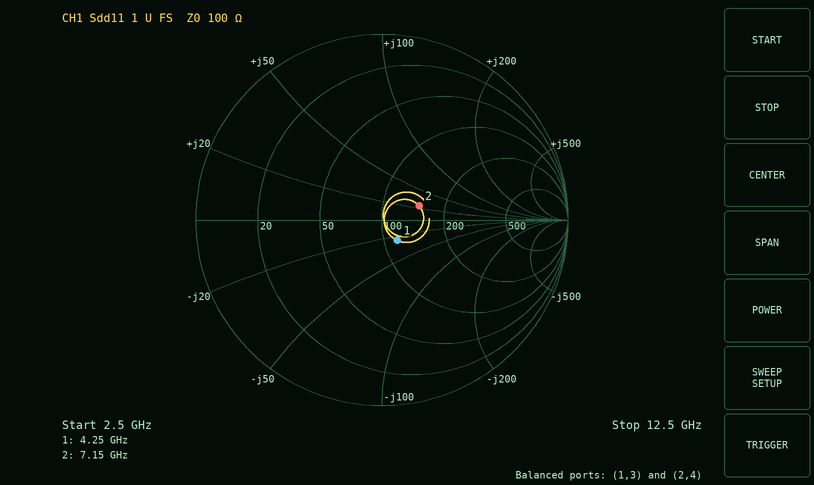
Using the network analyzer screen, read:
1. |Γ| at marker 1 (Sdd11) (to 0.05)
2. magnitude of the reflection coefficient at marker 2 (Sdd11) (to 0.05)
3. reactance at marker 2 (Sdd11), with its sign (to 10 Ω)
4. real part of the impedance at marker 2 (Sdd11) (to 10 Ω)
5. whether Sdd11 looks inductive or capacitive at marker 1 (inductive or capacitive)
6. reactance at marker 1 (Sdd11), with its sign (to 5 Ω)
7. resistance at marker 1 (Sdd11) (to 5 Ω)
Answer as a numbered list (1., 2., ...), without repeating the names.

1. 0.15
2. 0.20
3. +20 Ω
4. 150 Ω
5. capacitive
6. -25 Ω
7. 115 Ω
